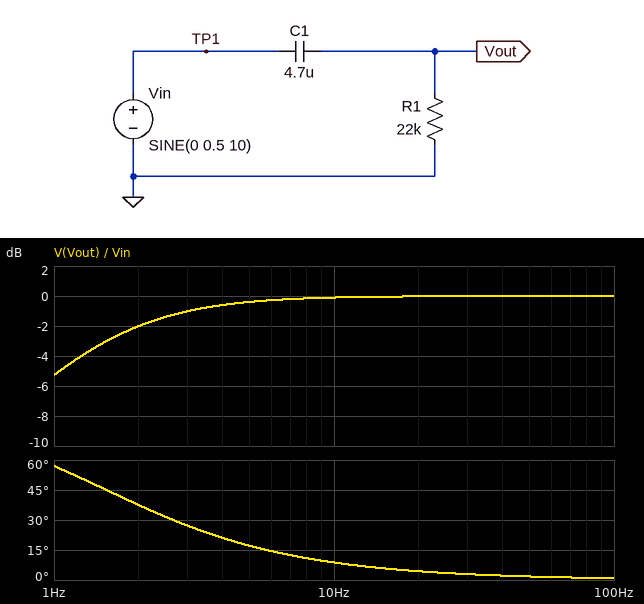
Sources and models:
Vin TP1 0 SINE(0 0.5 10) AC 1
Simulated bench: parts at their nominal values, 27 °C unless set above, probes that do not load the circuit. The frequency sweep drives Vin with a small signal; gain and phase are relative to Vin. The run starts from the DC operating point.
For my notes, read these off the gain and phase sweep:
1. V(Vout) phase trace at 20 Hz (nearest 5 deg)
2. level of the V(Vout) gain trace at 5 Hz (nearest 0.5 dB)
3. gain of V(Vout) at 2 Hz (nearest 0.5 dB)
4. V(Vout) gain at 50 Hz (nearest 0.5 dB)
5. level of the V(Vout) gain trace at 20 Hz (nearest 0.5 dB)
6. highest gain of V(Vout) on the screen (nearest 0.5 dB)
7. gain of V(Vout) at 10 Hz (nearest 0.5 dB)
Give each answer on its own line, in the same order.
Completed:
5 deg
-0.5 dB
-2.0 dB
0 dB
0 dB
0 dB
0 dB
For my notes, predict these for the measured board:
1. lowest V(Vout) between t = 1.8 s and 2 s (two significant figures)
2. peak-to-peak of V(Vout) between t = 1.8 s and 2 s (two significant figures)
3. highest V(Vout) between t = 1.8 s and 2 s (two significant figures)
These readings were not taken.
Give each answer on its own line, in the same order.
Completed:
-490 mV
990 mV
490 mV
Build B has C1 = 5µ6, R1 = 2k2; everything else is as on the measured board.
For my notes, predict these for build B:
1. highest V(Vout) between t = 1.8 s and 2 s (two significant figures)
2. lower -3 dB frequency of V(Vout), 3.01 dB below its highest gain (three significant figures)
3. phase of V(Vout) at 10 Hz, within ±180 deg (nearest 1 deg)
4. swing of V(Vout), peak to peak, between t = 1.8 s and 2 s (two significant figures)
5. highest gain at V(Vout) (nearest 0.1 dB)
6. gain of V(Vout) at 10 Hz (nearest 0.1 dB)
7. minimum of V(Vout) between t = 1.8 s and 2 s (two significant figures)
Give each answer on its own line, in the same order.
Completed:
310 mV
12.9 Hz
52 deg
610 mV
0 dB
-4.3 dB
-310 mV
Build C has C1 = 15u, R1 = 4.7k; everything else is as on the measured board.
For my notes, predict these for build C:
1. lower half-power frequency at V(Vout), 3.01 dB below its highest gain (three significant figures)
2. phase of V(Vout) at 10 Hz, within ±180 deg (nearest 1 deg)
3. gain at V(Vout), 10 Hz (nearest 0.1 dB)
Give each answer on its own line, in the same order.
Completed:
2.26 Hz
13 deg
-0.2 dB
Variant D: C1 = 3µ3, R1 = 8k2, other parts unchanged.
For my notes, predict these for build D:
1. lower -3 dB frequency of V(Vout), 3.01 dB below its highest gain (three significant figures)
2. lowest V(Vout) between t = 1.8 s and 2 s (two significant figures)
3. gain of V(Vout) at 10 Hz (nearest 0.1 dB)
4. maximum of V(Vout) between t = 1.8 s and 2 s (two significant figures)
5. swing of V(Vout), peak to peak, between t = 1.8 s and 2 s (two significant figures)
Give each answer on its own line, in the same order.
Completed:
5.88 Hz
-430 mV
-1.3 dB
430 mV
860 mV
